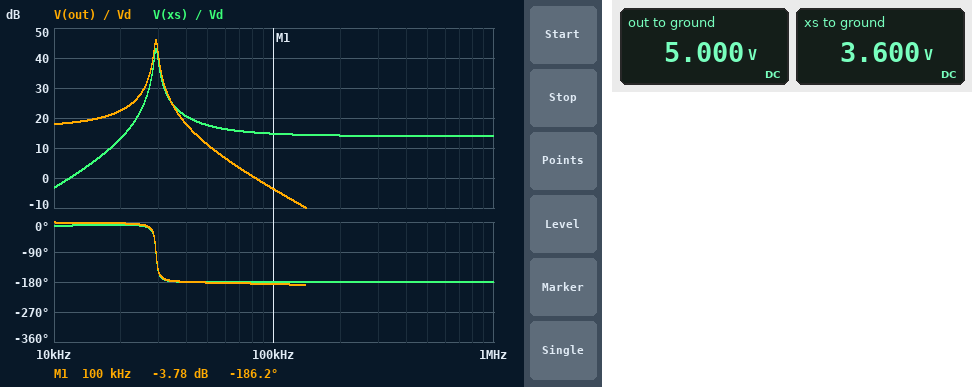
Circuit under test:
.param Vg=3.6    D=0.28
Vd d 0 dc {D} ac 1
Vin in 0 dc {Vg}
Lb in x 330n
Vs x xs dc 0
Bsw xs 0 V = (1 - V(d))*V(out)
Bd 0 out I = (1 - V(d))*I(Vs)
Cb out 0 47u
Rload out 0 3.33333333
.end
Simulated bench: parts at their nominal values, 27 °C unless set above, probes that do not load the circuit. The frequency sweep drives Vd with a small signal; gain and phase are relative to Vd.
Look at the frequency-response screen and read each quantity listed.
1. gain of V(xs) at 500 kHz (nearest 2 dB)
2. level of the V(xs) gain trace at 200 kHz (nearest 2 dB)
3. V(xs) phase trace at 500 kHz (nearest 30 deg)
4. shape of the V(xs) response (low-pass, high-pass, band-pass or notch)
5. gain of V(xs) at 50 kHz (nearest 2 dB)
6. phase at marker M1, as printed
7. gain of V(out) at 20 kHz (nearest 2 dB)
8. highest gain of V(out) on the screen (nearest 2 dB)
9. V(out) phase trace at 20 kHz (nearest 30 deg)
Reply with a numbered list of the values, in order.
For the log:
1. 14 dB
2. 14 dB
3. -180 deg
4. high-pass
5. 18 dB
6. -186.2 deg
7. 22 dB
8. 46 dB
9. 0 deg
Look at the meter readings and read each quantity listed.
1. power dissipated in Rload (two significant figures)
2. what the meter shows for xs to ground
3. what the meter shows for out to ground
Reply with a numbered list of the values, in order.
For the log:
1. 7.5 W
2. 3.600 V
3. 5.000 V
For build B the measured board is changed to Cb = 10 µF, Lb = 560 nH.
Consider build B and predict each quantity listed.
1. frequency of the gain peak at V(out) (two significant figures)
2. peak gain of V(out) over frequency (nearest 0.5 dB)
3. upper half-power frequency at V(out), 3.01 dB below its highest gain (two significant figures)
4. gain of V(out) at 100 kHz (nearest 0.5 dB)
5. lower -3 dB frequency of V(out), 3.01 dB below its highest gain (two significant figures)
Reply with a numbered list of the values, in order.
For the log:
1. 48 kHz
2. 37.0 dB
3. 51 kHz
4. 6.5 dB
5. 46 kHz
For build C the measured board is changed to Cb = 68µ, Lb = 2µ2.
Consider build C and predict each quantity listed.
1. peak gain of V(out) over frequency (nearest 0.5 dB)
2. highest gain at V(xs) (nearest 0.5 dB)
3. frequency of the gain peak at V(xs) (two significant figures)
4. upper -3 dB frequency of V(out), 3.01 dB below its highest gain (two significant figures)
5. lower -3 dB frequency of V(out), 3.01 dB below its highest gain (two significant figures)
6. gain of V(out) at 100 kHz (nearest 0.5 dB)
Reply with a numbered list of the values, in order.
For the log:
1. 39.5 dB
2. 36.5 dB
3. 9.4 kHz
4. 9.7 kHz
5. 9.0 kHz
6. -22.0 dB
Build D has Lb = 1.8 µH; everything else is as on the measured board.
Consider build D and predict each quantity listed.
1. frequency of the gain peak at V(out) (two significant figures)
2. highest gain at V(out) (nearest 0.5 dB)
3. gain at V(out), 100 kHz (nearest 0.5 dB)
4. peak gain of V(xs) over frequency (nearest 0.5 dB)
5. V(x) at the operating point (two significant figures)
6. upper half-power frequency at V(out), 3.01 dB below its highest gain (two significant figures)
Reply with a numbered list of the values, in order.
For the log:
1. 12 kHz
2. 38.5 dB
3. -17.5 dB
4. 36.0 dB
5. 3.6 V
6. 13 kHz
